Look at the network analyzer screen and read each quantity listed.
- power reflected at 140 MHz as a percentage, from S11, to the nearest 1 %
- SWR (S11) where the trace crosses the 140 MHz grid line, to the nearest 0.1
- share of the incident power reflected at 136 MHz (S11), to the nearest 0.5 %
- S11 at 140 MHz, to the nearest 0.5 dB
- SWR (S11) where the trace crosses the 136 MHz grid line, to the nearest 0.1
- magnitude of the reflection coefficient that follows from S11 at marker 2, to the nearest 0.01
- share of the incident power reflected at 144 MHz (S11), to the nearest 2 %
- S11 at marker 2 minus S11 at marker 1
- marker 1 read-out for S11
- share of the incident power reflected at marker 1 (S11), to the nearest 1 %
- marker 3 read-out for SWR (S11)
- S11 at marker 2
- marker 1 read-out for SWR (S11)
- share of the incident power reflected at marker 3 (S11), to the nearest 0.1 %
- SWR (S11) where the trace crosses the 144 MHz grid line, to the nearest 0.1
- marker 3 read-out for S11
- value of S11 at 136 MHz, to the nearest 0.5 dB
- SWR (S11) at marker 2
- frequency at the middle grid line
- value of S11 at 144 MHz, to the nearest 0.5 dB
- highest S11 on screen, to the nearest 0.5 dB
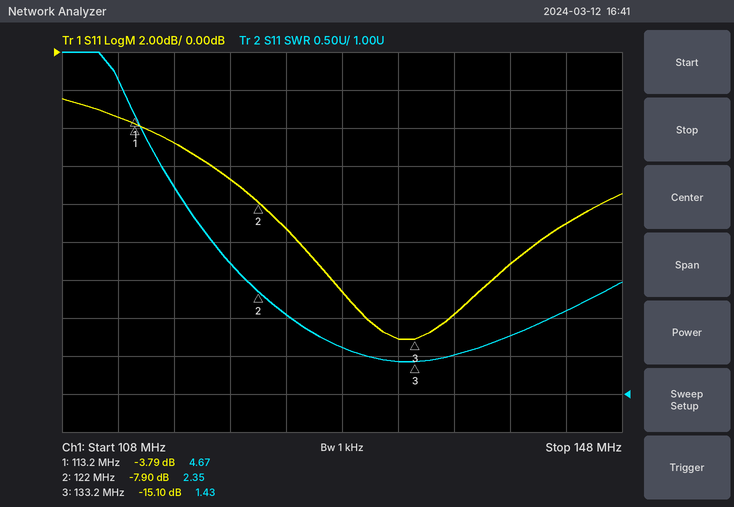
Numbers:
8 %
1.8
4.0 %
-11.0 dB
1.5
0.40
12 %
-4.11 dB
-3.79 dB
42 %
1.43
-7.90 dB
4.67
3.1 %
2.1
-15.10 dB
-14.0 dB
2.35
128 MHz
-9.0 dB
-2.5 dB
